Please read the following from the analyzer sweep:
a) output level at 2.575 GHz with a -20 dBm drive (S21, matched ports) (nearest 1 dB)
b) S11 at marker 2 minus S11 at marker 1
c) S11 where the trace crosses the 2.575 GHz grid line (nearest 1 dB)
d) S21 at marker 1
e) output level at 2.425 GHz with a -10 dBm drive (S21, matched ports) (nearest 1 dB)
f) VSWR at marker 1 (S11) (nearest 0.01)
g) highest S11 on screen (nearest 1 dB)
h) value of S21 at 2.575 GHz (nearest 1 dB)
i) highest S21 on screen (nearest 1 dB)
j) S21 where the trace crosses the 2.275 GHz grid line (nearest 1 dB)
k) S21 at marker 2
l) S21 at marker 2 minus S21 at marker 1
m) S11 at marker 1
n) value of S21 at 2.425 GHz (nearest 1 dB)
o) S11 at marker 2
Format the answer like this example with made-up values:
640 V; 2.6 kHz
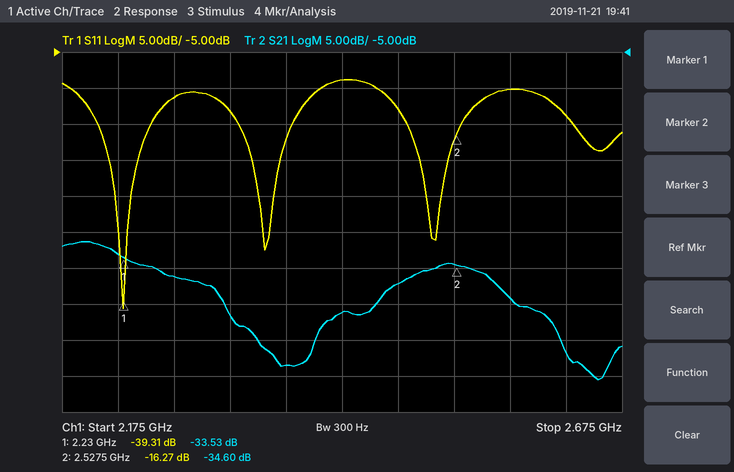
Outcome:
-59 dBm; 23.04 dB; -10 dB; -33.53 dB; -51 dBm; 1.02; -9 dB; -39 dB; -31 dB; -36 dB; -34.60 dB; -1.07 dB; -39.31 dB; -41 dB; -16.27 dB
